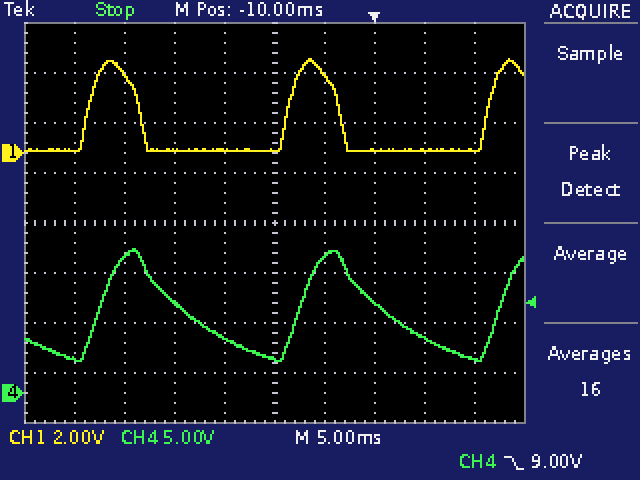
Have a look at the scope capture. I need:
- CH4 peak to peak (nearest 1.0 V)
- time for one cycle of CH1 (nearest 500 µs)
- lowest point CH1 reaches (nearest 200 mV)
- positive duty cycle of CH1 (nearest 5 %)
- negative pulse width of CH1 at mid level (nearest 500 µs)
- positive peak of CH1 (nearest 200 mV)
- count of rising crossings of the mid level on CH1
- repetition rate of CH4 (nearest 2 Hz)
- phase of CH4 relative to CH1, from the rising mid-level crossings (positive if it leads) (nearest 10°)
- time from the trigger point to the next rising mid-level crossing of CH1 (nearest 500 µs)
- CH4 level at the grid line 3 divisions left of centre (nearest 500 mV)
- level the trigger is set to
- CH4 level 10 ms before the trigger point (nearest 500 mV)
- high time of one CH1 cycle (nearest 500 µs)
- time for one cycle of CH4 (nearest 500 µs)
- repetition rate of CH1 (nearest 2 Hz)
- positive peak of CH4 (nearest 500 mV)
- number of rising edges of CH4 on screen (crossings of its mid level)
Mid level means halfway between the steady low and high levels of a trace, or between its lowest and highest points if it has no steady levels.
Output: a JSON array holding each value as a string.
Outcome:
["11.0 V", "20.0 ms", "0.0 V", "25 %", "15.0 ms", "3.8 V", "3", "50 Hz", "-20°", "11.5 ms", "13.5 V", "9.00 V", "3.5 V", "5.0 ms", "20.0 ms", "50 Hz", "14.5 V", "3"]
